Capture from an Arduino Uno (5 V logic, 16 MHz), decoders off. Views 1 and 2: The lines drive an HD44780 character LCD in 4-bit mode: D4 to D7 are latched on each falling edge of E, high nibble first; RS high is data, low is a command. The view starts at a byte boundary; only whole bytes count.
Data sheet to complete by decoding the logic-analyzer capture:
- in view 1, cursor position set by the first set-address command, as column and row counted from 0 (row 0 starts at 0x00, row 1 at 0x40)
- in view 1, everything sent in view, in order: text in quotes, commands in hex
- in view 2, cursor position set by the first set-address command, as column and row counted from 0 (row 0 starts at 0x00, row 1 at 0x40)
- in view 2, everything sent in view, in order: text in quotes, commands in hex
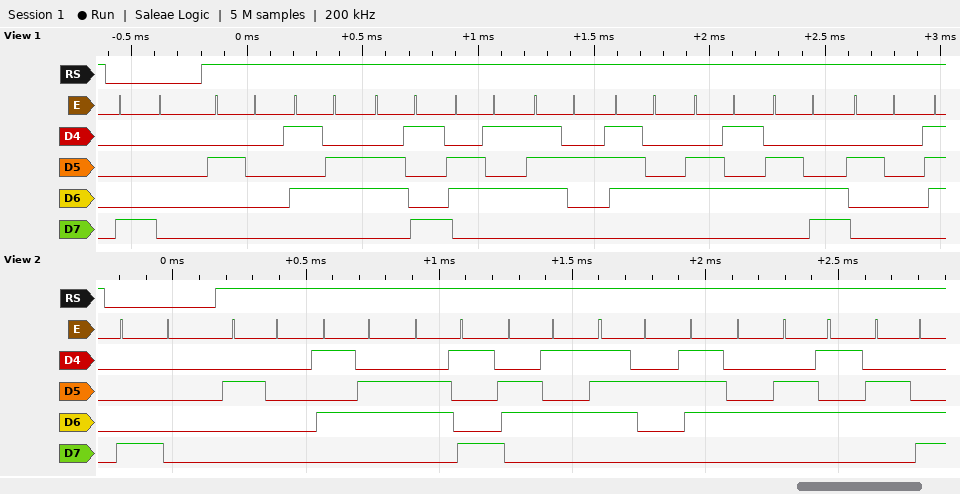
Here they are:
column 0, row 0
0x80 " Viertel "
column 0, row 0
0x80 " Viertel"
